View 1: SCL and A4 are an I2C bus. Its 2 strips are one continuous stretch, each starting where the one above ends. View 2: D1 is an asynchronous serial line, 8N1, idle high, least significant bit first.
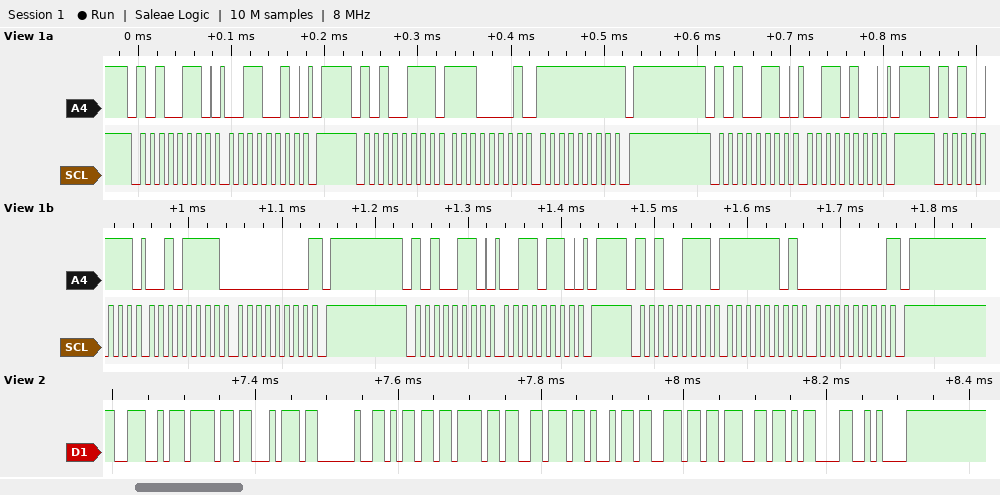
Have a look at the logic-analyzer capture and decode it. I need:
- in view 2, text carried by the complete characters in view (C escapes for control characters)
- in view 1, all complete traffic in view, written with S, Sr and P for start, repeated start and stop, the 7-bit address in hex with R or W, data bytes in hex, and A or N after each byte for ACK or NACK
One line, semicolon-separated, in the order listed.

"Not moving\r\n"; S 53W A 32 A P S 53R A E1 A FF N P S 53W A 34 A P S 53R A 2F A 00 N P S 53W A 36 A P S 53R A FD A 00 N P
